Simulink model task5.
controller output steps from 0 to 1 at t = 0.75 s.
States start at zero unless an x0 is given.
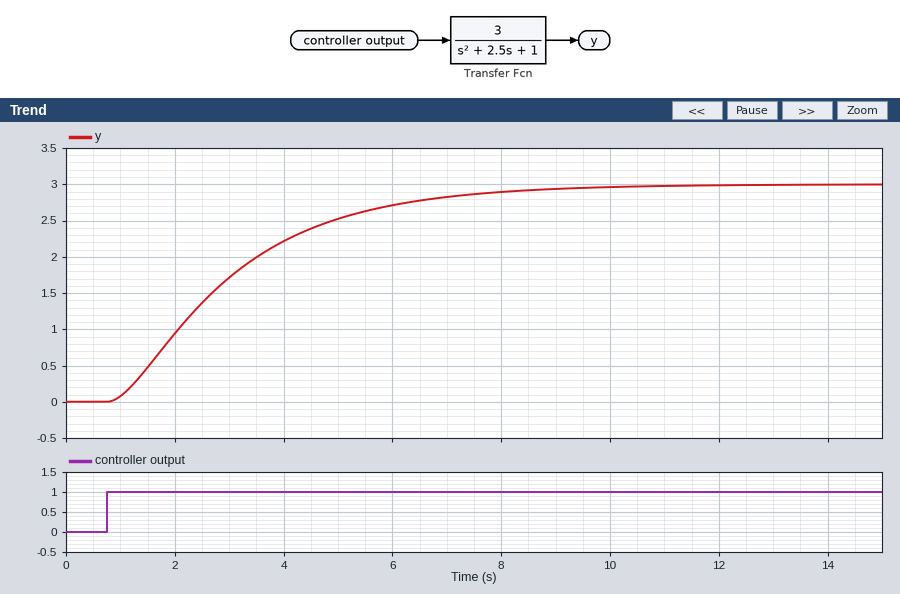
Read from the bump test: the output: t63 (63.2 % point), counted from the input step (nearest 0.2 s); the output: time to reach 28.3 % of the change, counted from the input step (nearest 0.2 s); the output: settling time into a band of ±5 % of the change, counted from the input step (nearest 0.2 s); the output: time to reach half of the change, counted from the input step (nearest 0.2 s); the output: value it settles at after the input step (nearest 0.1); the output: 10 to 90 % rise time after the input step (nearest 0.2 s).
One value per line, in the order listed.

2.6 s
1.2 s
6.6 s
2.0 s
3.0
4.6 s
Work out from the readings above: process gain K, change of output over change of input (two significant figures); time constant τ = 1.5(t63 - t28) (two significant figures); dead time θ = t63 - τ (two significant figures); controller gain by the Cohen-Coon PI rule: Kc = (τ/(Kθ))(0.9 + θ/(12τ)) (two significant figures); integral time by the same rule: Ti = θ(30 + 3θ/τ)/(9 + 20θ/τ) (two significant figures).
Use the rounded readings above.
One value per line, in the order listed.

3.0
2.1 s
0.50 s
1.3
1.1 s
